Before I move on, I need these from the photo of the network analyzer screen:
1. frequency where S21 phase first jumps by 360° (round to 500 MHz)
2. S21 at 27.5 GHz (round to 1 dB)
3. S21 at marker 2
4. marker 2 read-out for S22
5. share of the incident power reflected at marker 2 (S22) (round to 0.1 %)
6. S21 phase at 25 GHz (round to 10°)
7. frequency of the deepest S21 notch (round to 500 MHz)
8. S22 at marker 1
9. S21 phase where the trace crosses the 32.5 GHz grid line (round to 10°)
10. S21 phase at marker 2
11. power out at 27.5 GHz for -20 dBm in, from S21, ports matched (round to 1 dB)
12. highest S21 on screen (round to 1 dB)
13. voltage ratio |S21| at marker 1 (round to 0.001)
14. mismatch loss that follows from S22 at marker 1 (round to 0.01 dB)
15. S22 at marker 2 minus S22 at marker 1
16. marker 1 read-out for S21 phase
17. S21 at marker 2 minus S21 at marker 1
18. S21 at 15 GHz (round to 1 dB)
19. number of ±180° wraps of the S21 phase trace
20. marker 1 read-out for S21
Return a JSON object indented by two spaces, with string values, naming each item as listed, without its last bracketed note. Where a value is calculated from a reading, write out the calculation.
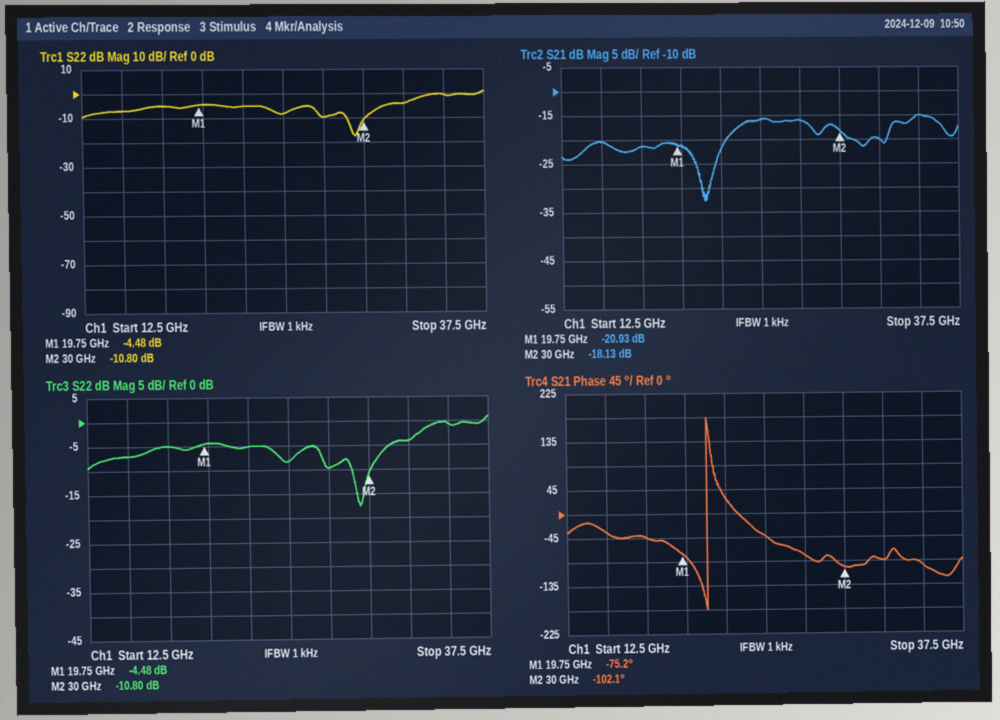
{
  "frequency where S21 phase first jumps by 360°": "21.5 GHz",
  "S21 at 27.5 GHz": "-16 dB",
  "S21 at marker 2": "-18.13 dB",
  "marker 2 read-out for S22": "-10.80 dB",
  "share of the incident power reflected at marker 2 (S22)": "10^(-10.8/10) ≈ 8.3 %",
  "S21 phase at 25 GHz": "-40°",
  "frequency of the deepest S21 notch": "21.5 GHz",
  "S22 at marker 1": "-4.48 dB",
  "S21 phase where the trace crosses the 32.5 GHz grid line": "-90°",
  "S21 phase at marker 2": "-102.1°",
  "power out at 27.5 GHz for -20 dBm in, from S21, ports matched": "-20 dBm + (-16 dB) = -36 dBm",
  "highest S21 on screen": "-15 dB",
  "voltage ratio |S21| at marker 1": "10^(-20.93/20) ≈ 0.090",
  "mismatch loss that follows from S22 at marker 1": "−10 log10(1 − 10^(-4.48/10)) ≈ 1.91 dB",
  "S22 at marker 2 minus S22 at marker 1": "-10.8 − (-4.48) = -6.32 dB",
  "marker 1 read-out for S21 phase": "-75.2°",
  "S21 at marker 2 minus S21 at marker 1": "-18.13 − (-20.93) = 2.80 dB",
  "S21 at 15 GHz": "-20 dB",
  "number of ±180° wraps of the S21 phase trace": "1",
  "marker 1 read-out for S21": "-20.93 dB"
}
